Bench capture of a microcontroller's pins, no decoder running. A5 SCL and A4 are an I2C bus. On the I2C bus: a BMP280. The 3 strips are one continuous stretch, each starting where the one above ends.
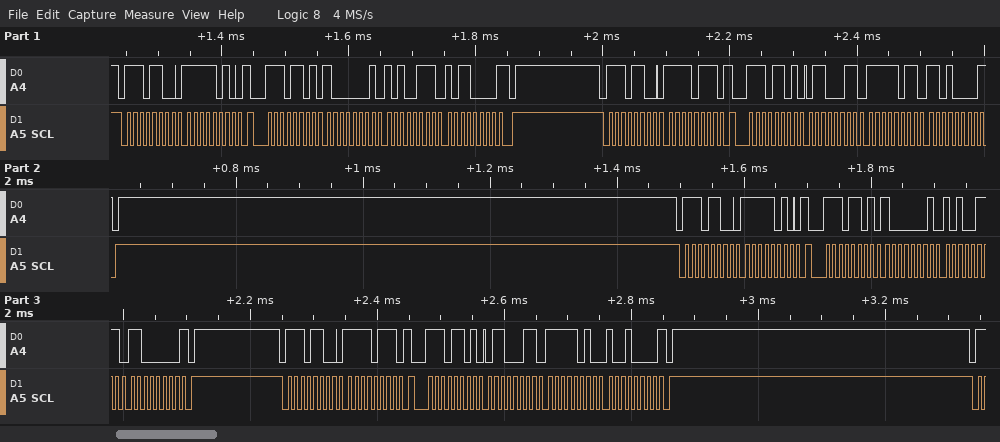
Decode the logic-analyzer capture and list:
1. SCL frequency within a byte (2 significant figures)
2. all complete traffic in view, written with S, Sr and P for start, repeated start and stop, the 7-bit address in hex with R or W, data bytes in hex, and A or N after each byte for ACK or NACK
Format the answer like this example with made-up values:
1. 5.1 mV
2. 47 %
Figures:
1. 100 kHz
2. S 76W A FA A Sr 76R A 81 A A7 A B0 N P S 76W A F7 A Sr 76R A 63 A FB A D0 N P S 76W A FA A Sr 76R A 81 A A7 A C0 N P S 76W A F7 A Sr 76R A 63 A FA A 90 N P
